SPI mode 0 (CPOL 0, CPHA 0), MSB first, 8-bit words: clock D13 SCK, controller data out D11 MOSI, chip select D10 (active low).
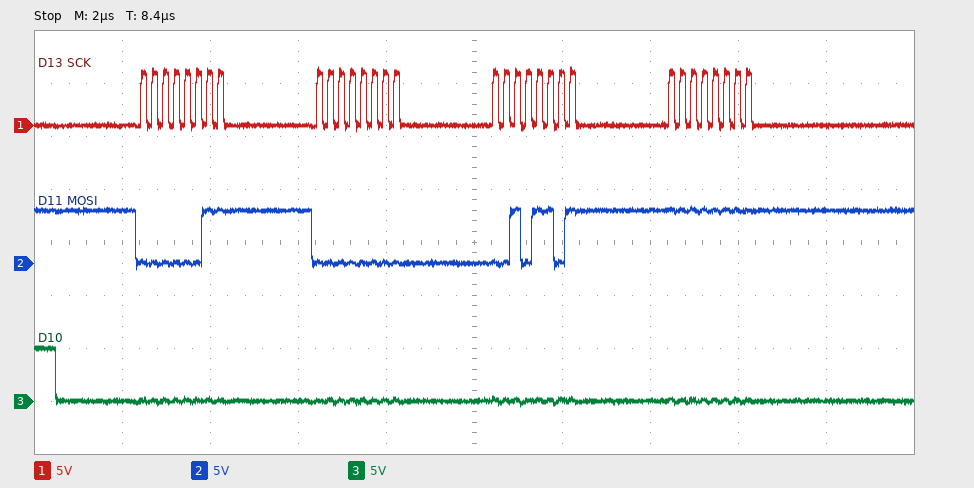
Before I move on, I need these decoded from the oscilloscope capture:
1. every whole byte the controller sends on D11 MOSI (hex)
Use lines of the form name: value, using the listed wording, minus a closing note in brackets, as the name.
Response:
every whole byte the controller sends on D11 MOSI: 03 00 2D FF
